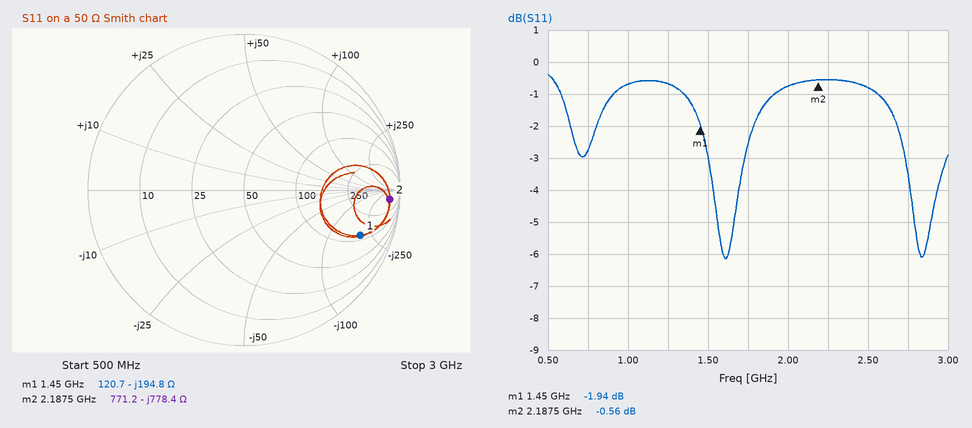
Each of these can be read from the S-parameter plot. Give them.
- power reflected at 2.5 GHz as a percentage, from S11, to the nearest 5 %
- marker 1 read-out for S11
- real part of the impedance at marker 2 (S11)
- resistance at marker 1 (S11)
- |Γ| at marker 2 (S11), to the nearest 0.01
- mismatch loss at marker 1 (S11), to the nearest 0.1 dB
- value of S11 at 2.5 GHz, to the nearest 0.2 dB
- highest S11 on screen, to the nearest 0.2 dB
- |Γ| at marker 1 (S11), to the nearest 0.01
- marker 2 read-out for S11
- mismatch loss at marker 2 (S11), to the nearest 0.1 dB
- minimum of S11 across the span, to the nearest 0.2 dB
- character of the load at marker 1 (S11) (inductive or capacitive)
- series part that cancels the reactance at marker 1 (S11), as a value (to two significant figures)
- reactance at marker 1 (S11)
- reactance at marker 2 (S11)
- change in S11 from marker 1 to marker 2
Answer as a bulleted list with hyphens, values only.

- 85 %
- -1.94 dB
- 771.2 Ω
- 120.7 Ω
- 0.94
- 4.4 dB
- -0.8 dB
- -0.4 dB
- 0.80
- -0.56 dB
- 9.2 dB
- -6.2 dB
- capacitive
- 21 nH
- -194.8 Ω
- -778.4 Ω
- 1.38 dB
